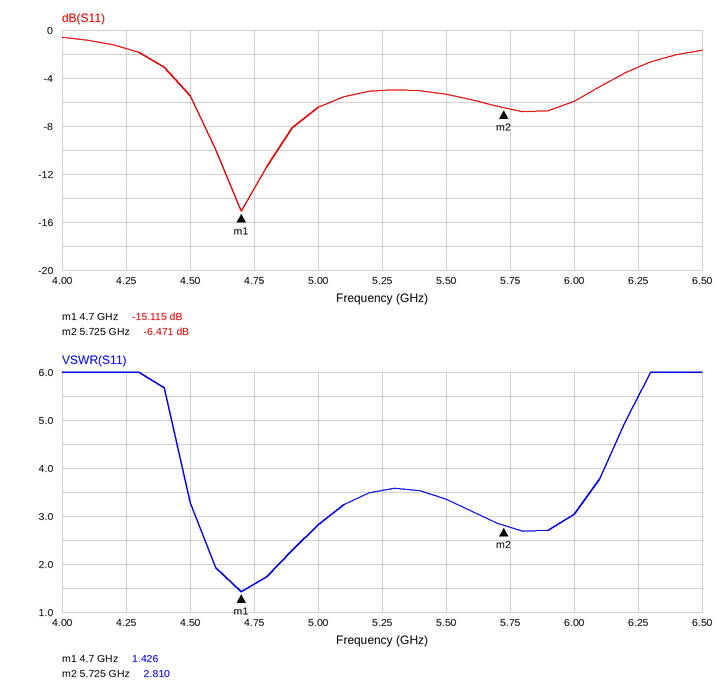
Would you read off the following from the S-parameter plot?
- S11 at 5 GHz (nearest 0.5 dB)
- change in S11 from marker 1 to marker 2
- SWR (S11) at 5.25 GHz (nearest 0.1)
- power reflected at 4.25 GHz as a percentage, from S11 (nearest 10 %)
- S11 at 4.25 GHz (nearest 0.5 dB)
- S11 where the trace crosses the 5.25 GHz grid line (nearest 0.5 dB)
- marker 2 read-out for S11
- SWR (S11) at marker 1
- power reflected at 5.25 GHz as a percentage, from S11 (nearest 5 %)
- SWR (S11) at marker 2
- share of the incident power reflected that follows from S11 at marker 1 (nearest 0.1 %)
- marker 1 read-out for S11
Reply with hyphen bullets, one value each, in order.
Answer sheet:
- -6.5 dB
- 8.644 dB
- 3.5
- 70 %
- -1.5 dB
- -5.0 dB
- -6.471 dB
- 1.426
- 30 %
- 2.810
- 3.1 %
- -15.115 dB
